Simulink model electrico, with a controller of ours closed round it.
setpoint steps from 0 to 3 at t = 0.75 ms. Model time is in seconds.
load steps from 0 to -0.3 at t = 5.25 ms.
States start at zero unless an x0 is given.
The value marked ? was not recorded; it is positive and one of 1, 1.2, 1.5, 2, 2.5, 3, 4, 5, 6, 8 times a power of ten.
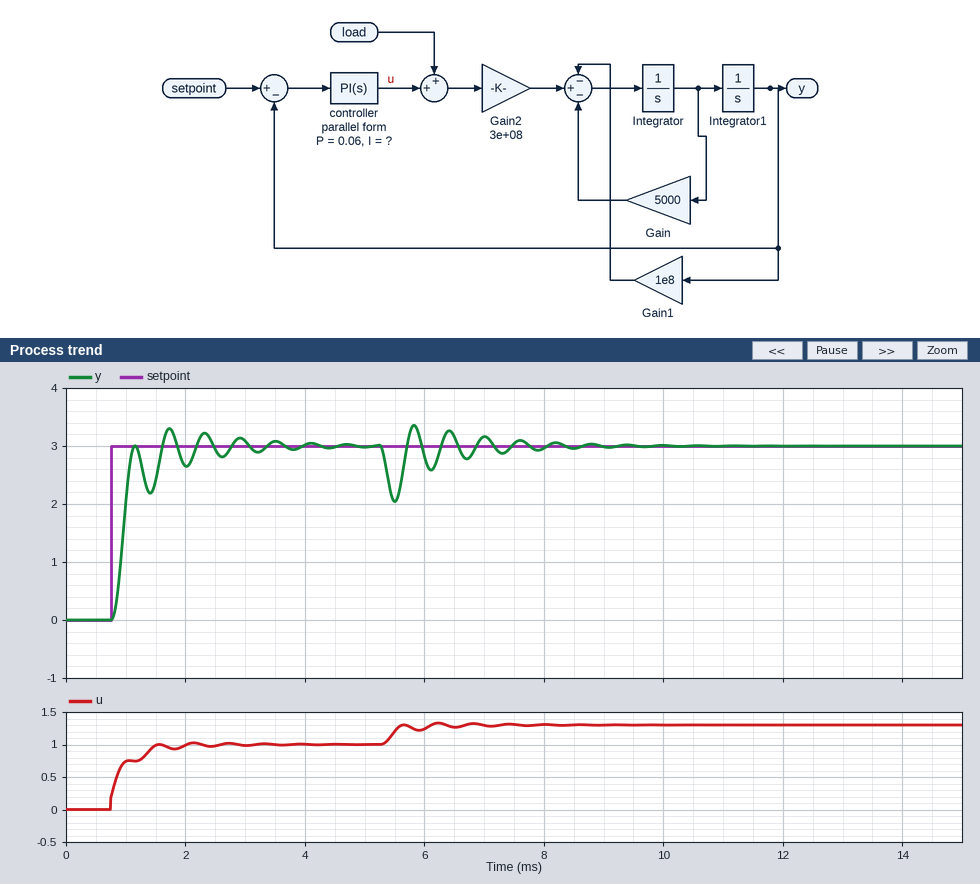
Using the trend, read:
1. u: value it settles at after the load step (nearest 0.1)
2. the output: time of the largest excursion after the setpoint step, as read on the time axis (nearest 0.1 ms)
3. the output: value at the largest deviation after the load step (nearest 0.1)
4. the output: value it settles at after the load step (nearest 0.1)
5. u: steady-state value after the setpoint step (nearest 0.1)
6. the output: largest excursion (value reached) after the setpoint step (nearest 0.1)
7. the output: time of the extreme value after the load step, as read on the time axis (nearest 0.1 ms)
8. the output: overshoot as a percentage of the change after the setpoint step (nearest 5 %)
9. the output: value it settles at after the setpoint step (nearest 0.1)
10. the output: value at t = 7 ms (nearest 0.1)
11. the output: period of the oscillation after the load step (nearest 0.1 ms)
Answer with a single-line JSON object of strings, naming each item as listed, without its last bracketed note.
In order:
{"u: value it settles at after the load step": "1.3", "the output: time of the largest excursion after the setpoint step, as read on the time axis": "1.7 ms", "the output: value at the largest deviation after the load step": "2.0", "the output: value it settles at after the load step": "3.0", "u: steady-state value after the setpoint step": "1.0", "the output: largest excursion (value reached) after the setpoint step": "3.3", "the output: time of the extreme value after the load step, as read on the time axis": "5.5 ms", "the output: overshoot as a percentage of the change after the setpoint step": "10 %", "the output: value it settles at after the setpoint step": "3.0", "the output: value at t = 7 ms": "3.2", "the output: period of the oscillation after the load step": "0.6 ms"}
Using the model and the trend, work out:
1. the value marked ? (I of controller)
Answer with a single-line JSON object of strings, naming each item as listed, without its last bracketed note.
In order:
{"the value marked ?": "1200"}
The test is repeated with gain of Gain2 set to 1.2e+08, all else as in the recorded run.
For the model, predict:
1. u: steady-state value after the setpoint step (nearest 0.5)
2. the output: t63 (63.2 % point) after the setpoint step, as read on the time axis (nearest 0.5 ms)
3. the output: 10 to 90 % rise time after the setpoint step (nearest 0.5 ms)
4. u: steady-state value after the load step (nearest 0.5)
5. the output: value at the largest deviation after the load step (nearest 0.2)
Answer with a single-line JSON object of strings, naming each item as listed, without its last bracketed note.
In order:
{"u: steady-state value after the setpoint step": "2.5", "the output: t63 (63.2 % point) after the setpoint step, as read on the time axis": "1.5 ms", "the output: 10 to 90 % rise time after the setpoint step": "1.5 ms", "u: steady-state value after the load step": "3.0", "the output: value at the largest deviation after the load step": "2.6"}
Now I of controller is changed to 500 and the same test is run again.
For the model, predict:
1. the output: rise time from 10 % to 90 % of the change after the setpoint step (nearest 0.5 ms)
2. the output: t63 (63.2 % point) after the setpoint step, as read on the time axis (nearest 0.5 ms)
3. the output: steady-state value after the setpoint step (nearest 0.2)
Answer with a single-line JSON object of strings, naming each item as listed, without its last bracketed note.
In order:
{"the output: rise time from 10 % to 90 % of the change after the setpoint step": "1.5 ms", "the output: t63 (63.2 % point) after the setpoint step, as read on the time axis": "1.5 ms", "the output: steady-state value after the setpoint step": "3.0"}
